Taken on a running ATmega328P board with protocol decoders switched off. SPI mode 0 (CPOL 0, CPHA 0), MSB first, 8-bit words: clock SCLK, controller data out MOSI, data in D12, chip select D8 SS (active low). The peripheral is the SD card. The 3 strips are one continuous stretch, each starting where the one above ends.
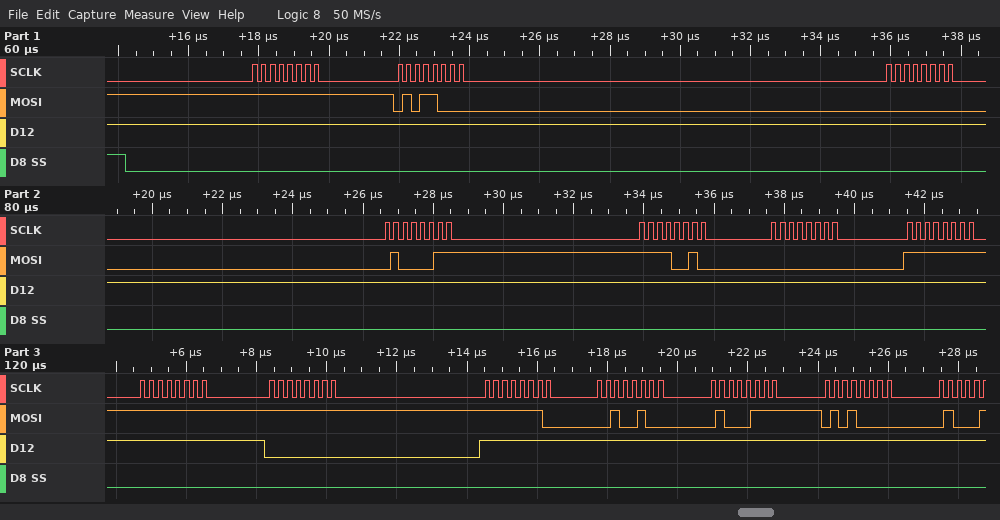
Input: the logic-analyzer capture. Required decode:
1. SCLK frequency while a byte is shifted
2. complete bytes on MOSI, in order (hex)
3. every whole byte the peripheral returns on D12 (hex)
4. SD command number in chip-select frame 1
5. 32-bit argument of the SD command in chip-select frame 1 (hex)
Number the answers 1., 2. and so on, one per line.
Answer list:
1. 4 MHz
2. FF 58 00 43 F2 00 FF FF FF FE 24 47 50
3. FF FF FF FF FF FF FF FF 00 FF FF FF FF
4. CMD24
5. 0x0043F200
